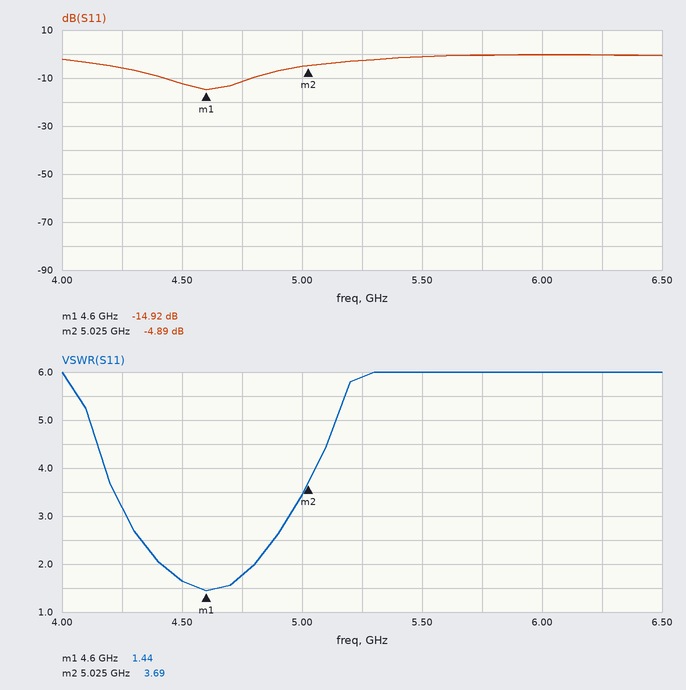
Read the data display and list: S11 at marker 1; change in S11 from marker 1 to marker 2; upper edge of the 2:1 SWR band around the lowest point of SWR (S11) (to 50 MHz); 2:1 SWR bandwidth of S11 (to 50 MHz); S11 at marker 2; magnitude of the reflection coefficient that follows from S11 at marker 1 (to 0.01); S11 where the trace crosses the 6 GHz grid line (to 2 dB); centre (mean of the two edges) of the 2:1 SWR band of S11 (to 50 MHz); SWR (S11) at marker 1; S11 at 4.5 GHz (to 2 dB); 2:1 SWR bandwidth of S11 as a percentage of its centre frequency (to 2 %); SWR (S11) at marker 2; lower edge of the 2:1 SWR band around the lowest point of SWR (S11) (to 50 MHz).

-14.92 dB
10.03 dB
4.80 GHz
400 MHz
-4.89 dB
0.18
0 dB
4.60 GHz
1.44
-12 dB
8 %
3.69
4.40 GHz
